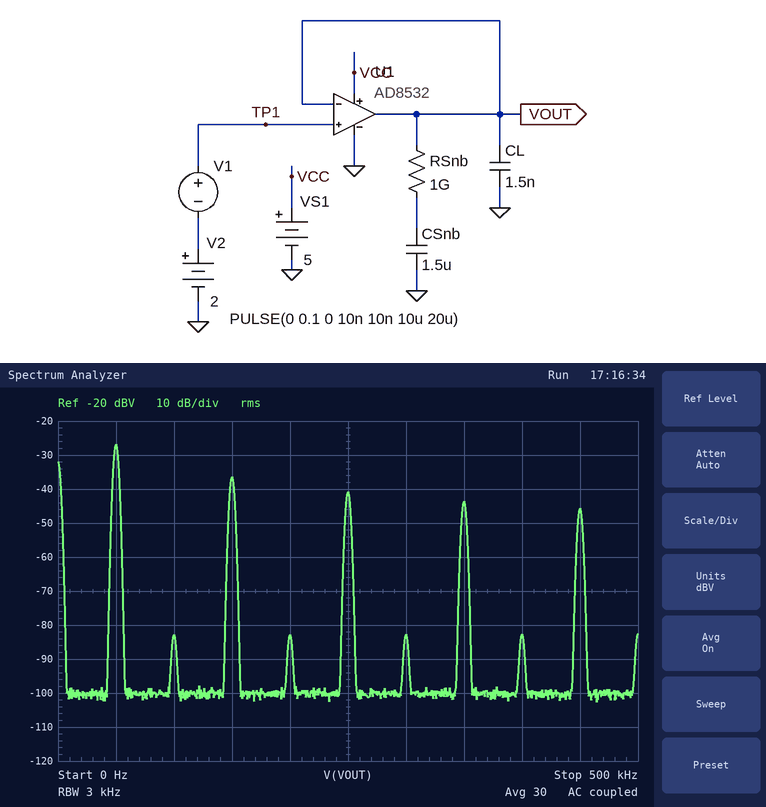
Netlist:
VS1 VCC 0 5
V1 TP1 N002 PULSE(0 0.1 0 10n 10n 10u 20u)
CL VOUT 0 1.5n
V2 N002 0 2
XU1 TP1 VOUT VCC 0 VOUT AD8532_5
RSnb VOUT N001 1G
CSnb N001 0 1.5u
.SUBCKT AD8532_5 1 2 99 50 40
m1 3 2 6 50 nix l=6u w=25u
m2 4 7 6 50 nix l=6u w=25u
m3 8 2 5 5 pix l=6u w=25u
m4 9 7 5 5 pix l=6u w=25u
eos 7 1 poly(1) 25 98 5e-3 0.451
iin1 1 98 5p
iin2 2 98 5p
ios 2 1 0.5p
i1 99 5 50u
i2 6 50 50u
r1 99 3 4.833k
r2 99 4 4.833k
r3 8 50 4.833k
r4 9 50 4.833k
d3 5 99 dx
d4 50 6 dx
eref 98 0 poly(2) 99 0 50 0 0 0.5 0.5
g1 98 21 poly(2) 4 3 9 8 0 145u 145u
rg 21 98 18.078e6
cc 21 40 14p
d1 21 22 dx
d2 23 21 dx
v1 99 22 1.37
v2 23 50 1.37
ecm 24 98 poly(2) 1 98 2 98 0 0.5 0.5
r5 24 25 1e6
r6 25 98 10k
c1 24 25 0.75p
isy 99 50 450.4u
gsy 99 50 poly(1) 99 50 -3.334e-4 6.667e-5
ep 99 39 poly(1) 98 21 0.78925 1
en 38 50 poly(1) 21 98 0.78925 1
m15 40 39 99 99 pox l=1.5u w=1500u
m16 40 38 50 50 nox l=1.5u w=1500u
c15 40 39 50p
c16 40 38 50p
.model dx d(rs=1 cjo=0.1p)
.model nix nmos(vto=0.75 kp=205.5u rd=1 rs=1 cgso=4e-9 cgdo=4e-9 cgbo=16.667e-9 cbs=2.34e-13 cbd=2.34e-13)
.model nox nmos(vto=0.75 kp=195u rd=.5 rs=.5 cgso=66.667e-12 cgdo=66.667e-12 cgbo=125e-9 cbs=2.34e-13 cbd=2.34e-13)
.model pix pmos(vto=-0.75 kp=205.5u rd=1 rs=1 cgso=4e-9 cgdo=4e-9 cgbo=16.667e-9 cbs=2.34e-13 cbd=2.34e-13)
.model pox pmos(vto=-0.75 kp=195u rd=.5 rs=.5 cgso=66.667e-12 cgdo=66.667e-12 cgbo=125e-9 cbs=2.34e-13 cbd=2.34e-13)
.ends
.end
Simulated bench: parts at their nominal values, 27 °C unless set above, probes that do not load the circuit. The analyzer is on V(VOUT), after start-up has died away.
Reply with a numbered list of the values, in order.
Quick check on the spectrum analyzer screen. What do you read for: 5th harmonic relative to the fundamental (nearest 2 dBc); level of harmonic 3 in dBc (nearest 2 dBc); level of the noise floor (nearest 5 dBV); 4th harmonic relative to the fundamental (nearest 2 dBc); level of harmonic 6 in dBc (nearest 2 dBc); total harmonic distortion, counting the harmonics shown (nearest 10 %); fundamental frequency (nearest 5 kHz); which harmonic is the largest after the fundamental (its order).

1. -14 dBc
2. -10 dBc
3. -100 dBV
4. -56 dBc
5. -56 dBc
6. 40 %
7. 50 kHz
8. 3
